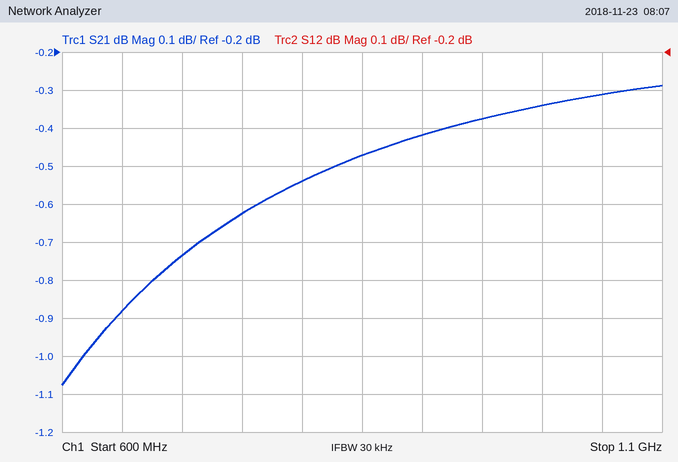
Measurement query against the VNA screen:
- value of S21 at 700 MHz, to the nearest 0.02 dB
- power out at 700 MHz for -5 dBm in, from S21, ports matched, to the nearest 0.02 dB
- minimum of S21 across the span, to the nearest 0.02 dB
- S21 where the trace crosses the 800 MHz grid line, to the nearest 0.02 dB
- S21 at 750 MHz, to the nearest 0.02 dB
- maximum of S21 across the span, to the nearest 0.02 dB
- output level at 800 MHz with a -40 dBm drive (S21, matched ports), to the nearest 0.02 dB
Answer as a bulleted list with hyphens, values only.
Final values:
- -0.74 dB
- -5.74 dBm
- -1.08 dB
- -0.54 dB
- -0.62 dB
- -0.28 dB
- -40.54 dBm
